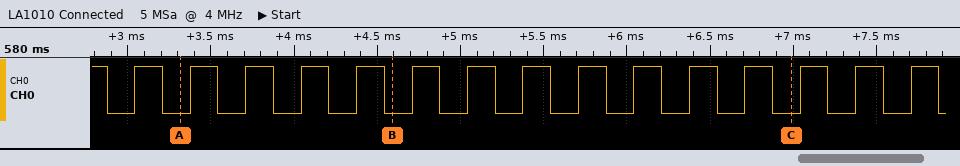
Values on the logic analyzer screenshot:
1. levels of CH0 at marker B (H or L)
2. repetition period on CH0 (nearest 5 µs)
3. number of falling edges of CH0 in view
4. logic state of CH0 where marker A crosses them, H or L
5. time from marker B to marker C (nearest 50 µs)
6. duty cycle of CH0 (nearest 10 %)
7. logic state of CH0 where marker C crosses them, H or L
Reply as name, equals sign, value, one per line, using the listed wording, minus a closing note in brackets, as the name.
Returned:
levels of CH0 at marker B = CH0=L
repetition period on CH0 = 335 µs
number of falling edges of CH0 in view = 16
logic state of CH0 where marker A crosses them, H or L = CH0=L
time from marker B to marker C = 2400 µs
duty cycle of CH0 = 50 %
logic state of CH0 where marker C crosses them, H or L = CH0=L
